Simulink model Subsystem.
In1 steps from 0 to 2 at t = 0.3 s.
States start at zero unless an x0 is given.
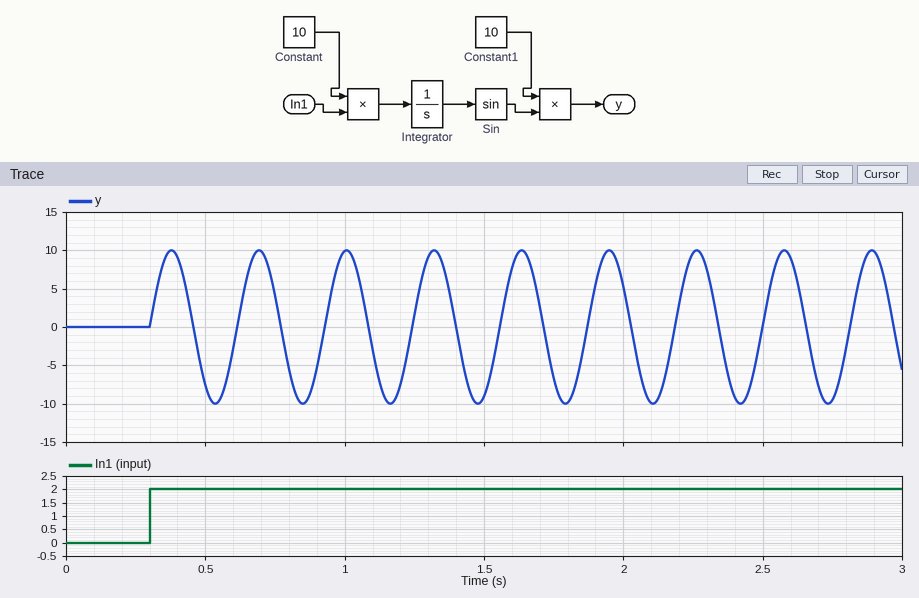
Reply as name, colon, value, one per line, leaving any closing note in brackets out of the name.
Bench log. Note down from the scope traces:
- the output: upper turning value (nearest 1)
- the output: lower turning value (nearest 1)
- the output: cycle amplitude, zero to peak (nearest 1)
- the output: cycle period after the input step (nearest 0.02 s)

the output: upper turning value: 10
the output: lower turning value: -10
the output: cycle amplitude, zero to peak: 10
the output: cycle period after the input step: 0.32 s
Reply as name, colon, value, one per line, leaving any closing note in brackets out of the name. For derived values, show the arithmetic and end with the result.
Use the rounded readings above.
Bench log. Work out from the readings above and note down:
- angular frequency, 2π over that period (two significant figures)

angular frequency, 2π over that period: 2π / 0.32 = 20 rad/s
